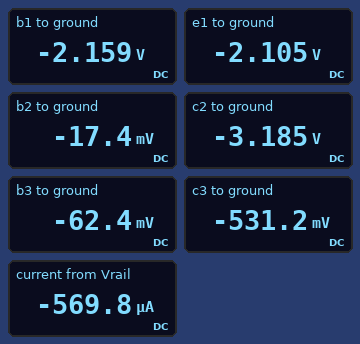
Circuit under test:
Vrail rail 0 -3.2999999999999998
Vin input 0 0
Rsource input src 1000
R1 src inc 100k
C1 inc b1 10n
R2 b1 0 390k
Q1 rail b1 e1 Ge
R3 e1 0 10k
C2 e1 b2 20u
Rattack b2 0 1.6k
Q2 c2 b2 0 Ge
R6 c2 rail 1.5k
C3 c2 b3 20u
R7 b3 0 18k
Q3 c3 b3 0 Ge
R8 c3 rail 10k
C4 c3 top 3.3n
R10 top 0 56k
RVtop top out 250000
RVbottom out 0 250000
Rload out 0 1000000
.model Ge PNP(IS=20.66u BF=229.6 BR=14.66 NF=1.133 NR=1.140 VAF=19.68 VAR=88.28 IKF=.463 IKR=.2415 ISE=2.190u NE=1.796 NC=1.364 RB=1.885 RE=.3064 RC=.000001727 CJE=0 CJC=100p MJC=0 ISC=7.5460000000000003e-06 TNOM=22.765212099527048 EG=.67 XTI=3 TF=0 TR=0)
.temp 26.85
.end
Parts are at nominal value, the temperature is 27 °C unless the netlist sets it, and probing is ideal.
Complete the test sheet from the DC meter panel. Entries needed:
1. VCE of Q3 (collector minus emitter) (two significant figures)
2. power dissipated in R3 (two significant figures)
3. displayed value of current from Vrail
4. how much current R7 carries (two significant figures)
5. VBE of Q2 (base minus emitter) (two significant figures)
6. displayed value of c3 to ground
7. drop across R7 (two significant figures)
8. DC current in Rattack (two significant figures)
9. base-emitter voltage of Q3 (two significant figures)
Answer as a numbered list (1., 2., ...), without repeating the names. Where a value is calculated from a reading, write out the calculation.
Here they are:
1. -531.2 mV = -530 mV
2. (0 V - (-2.105 V))^2 / 10 kΩ = 440 µW
3. -569.8 µA
4. (0 V - (-62.4 mV)) / 18 kΩ = 3.5 µA
5. -17.4 mV = -17 mV
6. -531.2 mV
7. 0 V - (-62.4 mV) = 62 mV
8. (0 V - (-17.4 mV)) / 1.6 kΩ = 11 µA
9. -62.4 mV = -62 mV
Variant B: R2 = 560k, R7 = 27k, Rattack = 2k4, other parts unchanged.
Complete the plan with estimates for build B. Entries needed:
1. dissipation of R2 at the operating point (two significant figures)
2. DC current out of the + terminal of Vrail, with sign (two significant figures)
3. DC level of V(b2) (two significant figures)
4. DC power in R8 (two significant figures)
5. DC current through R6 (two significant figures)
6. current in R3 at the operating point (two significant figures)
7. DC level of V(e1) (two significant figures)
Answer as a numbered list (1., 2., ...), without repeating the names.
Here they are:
1. 11 µW
2. -650 µA
3. -24 mV
4. 930 µW
5. 94 µA
6. 240 µA
7. -2.4 V
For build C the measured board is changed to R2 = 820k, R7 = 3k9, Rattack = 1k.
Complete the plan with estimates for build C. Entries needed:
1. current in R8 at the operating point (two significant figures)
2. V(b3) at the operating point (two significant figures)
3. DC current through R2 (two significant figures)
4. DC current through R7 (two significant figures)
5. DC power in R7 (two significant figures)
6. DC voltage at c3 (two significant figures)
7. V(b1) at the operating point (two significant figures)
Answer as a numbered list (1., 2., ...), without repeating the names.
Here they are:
1. 120 µA
2. -35 mV
3. 3.4 µA
4. 8.9 µA
5. 310 nW
6. -2.1 V
7. -2.8 V
